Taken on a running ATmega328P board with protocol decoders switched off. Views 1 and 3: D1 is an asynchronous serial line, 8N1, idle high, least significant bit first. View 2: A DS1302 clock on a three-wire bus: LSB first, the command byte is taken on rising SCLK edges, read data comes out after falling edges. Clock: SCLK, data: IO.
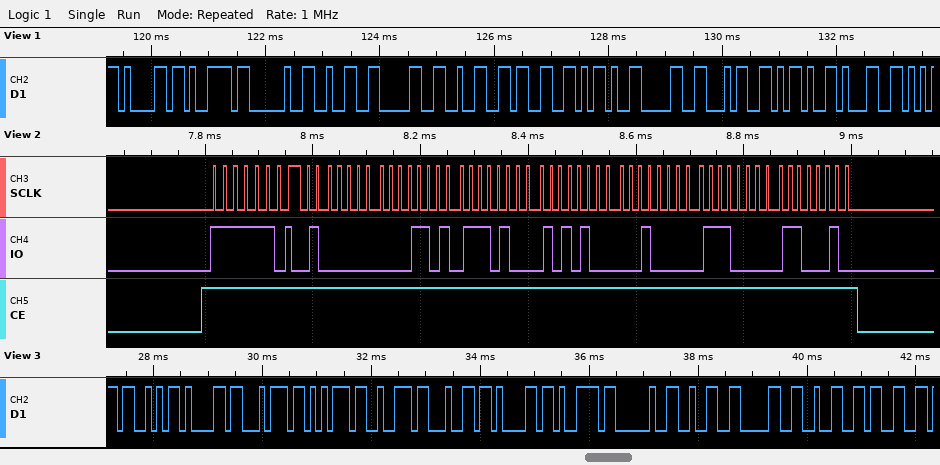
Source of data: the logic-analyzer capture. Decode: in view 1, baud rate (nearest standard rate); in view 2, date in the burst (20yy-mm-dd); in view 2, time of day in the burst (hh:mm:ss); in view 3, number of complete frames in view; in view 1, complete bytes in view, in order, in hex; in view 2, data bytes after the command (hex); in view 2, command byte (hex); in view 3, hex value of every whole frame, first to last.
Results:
9600 baud
2023-04-15
17:58:02
13
61 79 20 32 30 32 33 2D 30 34 2D 31
02 58 17 15 04 07 23
0xBF
53 61 74 75 72 64 61 79 20 32 30 32 33
